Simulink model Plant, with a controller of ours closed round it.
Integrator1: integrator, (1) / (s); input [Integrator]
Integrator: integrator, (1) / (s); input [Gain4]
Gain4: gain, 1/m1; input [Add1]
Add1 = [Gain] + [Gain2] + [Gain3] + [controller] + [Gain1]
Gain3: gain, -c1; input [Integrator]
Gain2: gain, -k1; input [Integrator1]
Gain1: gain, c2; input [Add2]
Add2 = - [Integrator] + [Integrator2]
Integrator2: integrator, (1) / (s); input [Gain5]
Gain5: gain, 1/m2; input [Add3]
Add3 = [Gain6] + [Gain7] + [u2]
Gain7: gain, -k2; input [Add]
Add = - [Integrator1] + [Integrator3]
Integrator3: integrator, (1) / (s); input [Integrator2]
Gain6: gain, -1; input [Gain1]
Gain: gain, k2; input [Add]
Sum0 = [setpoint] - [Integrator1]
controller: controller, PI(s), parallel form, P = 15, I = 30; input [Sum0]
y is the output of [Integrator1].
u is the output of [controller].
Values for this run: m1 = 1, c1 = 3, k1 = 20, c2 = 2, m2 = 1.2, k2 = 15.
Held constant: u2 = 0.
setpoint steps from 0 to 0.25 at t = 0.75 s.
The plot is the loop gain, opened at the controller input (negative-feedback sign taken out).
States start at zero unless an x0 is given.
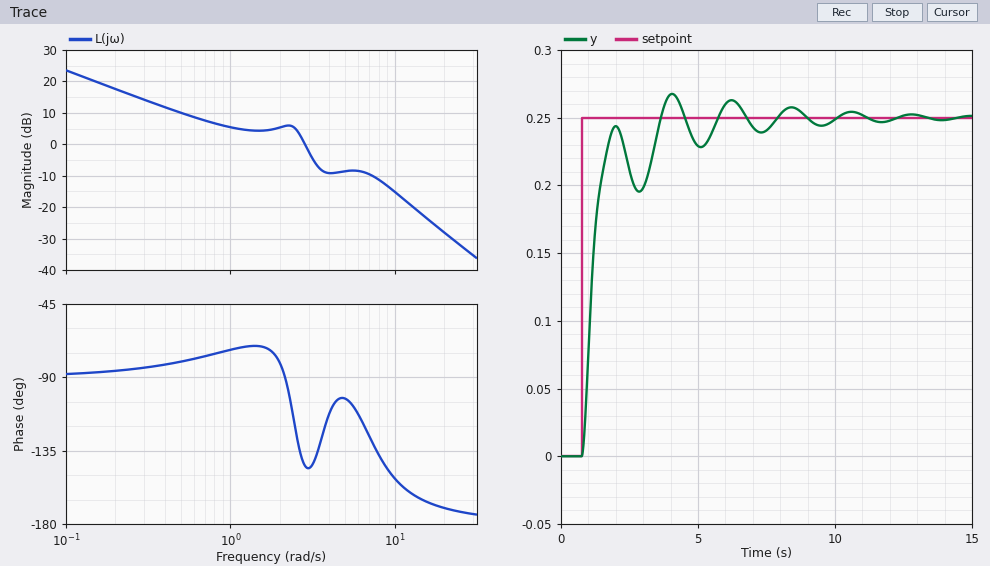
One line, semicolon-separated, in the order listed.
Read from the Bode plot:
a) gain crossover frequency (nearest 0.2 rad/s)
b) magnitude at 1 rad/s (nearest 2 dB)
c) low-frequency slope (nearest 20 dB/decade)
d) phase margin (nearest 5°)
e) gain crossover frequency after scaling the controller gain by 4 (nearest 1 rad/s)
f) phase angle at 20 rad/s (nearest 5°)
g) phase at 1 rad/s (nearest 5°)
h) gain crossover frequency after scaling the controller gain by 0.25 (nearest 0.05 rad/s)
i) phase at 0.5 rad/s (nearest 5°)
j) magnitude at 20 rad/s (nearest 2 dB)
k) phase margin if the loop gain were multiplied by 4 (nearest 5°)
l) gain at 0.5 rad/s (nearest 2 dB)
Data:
2.8 rad/s; 6 dB; -20 dB/decade; 35°; 8 rad/s; -170°; -75°; 0.40 rad/s; -80°; -28 dB; 40°; 10 dB
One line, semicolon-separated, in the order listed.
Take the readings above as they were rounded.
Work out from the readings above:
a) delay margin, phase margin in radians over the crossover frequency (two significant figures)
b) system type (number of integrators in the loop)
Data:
0.22 s; 1
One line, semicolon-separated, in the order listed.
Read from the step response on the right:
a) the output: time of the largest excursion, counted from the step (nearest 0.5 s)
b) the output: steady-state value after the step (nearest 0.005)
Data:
3.5 s; 0.250
